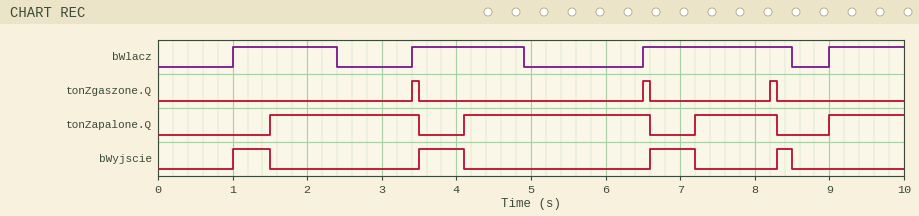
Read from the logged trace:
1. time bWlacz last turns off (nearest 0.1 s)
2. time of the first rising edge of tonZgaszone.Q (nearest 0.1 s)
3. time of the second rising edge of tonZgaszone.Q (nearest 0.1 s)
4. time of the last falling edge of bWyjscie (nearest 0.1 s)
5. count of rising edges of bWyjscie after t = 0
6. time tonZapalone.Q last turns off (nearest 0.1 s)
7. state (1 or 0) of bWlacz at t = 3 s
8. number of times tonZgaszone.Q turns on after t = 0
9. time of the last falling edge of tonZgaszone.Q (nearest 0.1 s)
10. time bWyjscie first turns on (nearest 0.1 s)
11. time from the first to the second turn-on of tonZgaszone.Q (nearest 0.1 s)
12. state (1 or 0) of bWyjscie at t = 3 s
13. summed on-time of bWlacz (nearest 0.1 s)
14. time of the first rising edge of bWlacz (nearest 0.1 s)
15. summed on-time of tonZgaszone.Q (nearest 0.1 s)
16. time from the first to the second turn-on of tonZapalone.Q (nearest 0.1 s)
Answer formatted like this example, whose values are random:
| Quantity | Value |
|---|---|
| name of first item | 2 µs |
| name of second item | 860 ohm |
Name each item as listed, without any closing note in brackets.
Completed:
| Quantity | Value |
|---|---|
| time bWlacz last turns off | 8.5 s |
| time of the first rising edge of tonZgaszone.Q | 3.4 s |
| time of the second rising edge of tonZgaszone.Q | 6.5 s |
| time of the last falling edge of bWyjscie | 8.5 s |
| count of rising edges of bWyjscie after t = 0 | 4 |
| time tonZapalone.Q last turns off | 8.3 s |
| state (1 or 0) of bWlacz at t = 3 s | 0 |
| number of times tonZgaszone.Q turns on after t = 0 | 3 |
| time of the last falling edge of tonZgaszone.Q | 8.3 s |
| time bWyjscie first turns on | 1.0 s |
| time from the first to the second turn-on of tonZgaszone.Q | 3.1 s |
| state (1 or 0) of bWyjscie at t = 3 s | 0 |
| summed on-time of bWlacz | 5.9 s |
| time of the first rising edge of bWlacz | 1.0 s |
| summed on-time of tonZgaszone.Q | 0.3 s |
| time from the first to the second turn-on of tonZapalone.Q | 2.6 s |
